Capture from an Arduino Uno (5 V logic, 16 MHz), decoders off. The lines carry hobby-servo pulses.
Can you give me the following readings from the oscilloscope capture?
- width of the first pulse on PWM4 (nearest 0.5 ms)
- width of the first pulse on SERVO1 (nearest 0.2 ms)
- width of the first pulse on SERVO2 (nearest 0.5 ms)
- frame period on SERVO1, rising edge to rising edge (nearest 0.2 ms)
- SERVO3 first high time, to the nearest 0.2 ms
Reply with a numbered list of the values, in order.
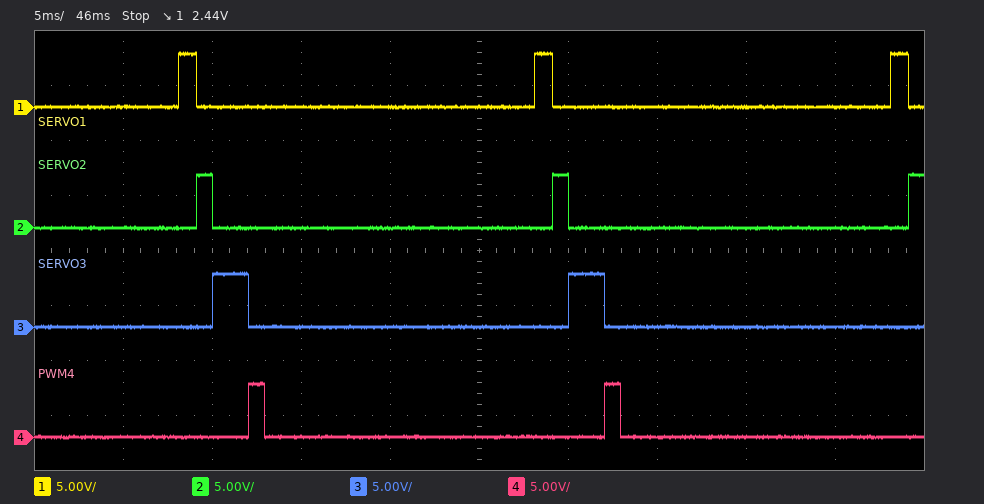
1. 1.0 ms
2. 1.0 ms
3. 1.0 ms
4. 20.0 ms
5. 2.0 ms
